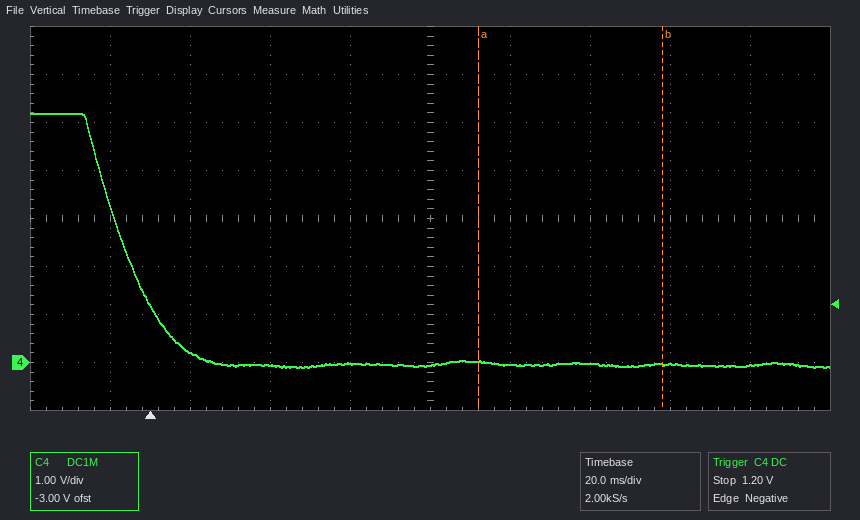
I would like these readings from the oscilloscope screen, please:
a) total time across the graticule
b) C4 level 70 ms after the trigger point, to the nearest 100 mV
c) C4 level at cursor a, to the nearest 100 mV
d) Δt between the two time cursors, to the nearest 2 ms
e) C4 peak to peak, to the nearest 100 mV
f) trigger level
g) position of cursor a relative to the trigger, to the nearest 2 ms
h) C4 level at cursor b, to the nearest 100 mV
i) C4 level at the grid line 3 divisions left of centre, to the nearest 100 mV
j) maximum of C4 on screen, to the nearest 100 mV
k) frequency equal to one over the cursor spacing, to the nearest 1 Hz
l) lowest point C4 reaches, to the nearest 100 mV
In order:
200 ms
-100 mV
0.0 V
46 ms
5.3 V
1.20 V
+82 ms
0.0 V
200 mV
5.2 V
22 Hz
-100 mV
